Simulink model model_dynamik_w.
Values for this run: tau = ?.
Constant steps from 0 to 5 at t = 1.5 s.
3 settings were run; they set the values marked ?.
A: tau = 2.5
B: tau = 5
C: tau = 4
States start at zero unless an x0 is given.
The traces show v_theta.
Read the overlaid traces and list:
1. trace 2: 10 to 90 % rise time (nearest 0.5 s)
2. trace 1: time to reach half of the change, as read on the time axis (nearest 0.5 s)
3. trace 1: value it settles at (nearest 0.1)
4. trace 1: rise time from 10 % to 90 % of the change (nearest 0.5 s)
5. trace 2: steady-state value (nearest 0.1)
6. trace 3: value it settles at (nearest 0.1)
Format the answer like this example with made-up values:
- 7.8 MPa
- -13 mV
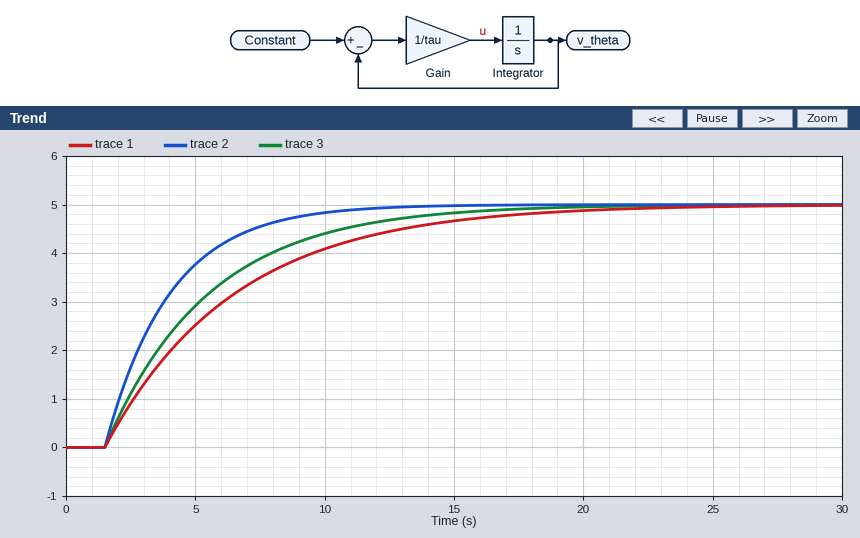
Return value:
- 5.5 s
- 5.0 s
- 5.0
- 11.0 s
- 5.0
- 5.0
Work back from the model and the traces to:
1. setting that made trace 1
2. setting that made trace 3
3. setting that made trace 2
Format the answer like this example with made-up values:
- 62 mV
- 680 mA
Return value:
- B
- C
- A
